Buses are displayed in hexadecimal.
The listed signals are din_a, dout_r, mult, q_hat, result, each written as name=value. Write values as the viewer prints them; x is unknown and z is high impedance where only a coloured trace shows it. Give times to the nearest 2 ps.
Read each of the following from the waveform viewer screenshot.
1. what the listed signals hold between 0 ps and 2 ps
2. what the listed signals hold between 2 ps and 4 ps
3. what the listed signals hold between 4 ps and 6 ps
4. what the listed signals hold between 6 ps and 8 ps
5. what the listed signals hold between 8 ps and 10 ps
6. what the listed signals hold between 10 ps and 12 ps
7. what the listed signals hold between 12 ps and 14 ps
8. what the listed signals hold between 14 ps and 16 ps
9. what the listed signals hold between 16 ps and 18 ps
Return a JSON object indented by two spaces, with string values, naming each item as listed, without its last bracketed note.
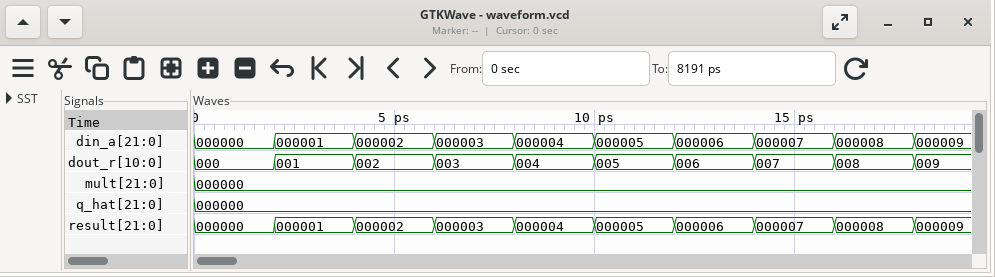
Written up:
{
  "what the listed signals hold between 0 ps and 2 ps": "din_a=000000, dout_r=000, mult=000000, q_hat=000000, result=000000",
  "what the listed signals hold between 2 ps and 4 ps": "din_a=000001, dout_r=001, mult=000000, q_hat=000000, result=000001",
  "what the listed signals hold between 4 ps and 6 ps": "din_a=000002, dout_r=002, mult=000000, q_hat=000000, result=000002",
  "what the listed signals hold between 6 ps and 8 ps": "din_a=000003, dout_r=003, mult=000000, q_hat=000000, result=000003",
  "what the listed signals hold between 8 ps and 10 ps": "din_a=000004, dout_r=004, mult=000000, q_hat=000000, result=000004",
  "what the listed signals hold between 10 ps and 12 ps": "din_a=000005, dout_r=005, mult=000000, q_hat=000000, result=000005",
  "what the listed signals hold between 12 ps and 14 ps": "din_a=000006, dout_r=006, mult=000000, q_hat=000000, result=000006",
  "what the listed signals hold between 14 ps and 16 ps": "din_a=000007, dout_r=007, mult=000000, q_hat=000000, result=000007",
  "what the listed signals hold between 16 ps and 18 ps": "din_a=000008, dout_r=008, mult=000000, q_hat=000000, result=000008"
}
